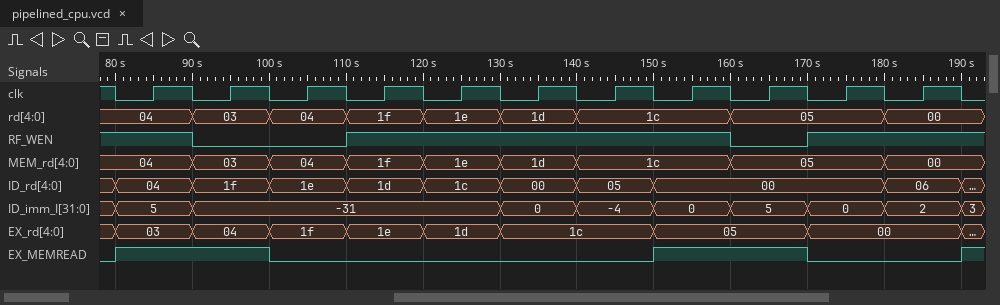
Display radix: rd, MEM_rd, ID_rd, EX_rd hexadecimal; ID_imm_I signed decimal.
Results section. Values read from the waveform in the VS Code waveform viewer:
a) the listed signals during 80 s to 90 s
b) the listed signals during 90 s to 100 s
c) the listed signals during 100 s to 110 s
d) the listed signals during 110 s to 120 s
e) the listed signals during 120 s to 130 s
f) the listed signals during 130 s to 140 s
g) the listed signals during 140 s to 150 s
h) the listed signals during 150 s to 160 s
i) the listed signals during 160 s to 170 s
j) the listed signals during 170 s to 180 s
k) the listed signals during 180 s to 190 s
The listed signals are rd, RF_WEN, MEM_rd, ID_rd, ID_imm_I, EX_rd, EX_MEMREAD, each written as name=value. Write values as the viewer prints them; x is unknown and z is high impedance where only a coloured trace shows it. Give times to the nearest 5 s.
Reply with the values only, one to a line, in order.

rd=04, RF_WEN=1, MEM_rd=04, ID_rd=04, ID_imm_I=5, EX_rd=03, EX_MEMREAD=1
rd=03, RF_WEN=0, MEM_rd=03, ID_rd=1f, ID_imm_I=-31, EX_rd=04, EX_MEMREAD=1
rd=04, RF_WEN=0, MEM_rd=04, ID_rd=1e, ID_imm_I=-31, EX_rd=1f, EX_MEMREAD=0
rd=1f, RF_WEN=1, MEM_rd=1f, ID_rd=1d, ID_imm_I=-31, EX_rd=1e, EX_MEMREAD=0
rd=1e, RF_WEN=1, MEM_rd=1e, ID_rd=1c, ID_imm_I=-31, EX_rd=1d, EX_MEMREAD=0
rd=1d, RF_WEN=1, MEM_rd=1d, ID_rd=00, ID_imm_I=0, EX_rd=1c, EX_MEMREAD=0
rd=1c, RF_WEN=1, MEM_rd=1c, ID_rd=05, ID_imm_I=-4, EX_rd=1c, EX_MEMREAD=0
rd=1c, RF_WEN=1, MEM_rd=1c, ID_rd=00, ID_imm_I=0, EX_rd=05, EX_MEMREAD=1
rd=05, RF_WEN=0, MEM_rd=05, ID_rd=00, ID_imm_I=5, EX_rd=05, EX_MEMREAD=1
rd=05, RF_WEN=1, MEM_rd=05, ID_rd=00, ID_imm_I=0, EX_rd=00, EX_MEMREAD=0
rd=00, RF_WEN=1, MEM_rd=00, ID_rd=06, ID_imm_I=2, EX_rd=00, EX_MEMREAD=0
